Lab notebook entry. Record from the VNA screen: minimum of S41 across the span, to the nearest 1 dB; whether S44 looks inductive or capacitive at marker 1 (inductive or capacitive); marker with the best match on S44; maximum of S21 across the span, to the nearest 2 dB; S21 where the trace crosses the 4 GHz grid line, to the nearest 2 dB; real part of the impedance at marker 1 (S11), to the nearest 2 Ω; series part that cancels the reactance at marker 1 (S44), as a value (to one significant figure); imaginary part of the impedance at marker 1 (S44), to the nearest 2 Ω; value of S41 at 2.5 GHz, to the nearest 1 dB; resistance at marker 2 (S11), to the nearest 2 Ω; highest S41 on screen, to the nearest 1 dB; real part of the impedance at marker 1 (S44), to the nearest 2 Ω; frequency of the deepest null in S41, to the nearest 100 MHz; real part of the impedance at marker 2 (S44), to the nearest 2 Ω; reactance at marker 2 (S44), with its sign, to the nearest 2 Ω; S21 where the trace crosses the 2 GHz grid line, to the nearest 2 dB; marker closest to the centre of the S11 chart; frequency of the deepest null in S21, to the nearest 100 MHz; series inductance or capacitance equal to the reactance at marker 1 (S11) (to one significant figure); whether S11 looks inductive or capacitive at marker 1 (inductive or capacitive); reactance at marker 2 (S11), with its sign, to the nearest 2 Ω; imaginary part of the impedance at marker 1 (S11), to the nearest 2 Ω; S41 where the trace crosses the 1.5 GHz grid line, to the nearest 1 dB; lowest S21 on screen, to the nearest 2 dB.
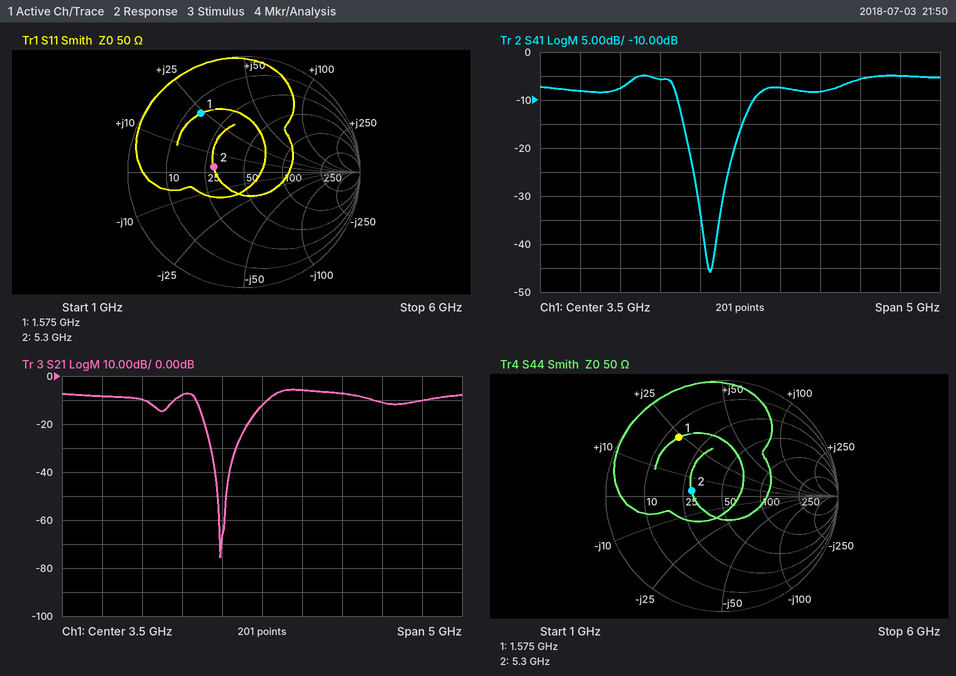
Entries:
-46 dB
inductive
marker 2
-6 dB
-6 dB
14 Ω
4 pF
+24 Ω
-6 dB
30 Ω
-5 dB
14 Ω
3.1 GHz
30 Ω
+2 Ω
-10 dB
marker 2
3.0 GHz
2 nH
inductive
+2 Ω
+24 Ω
-8 dB
-76 dB
